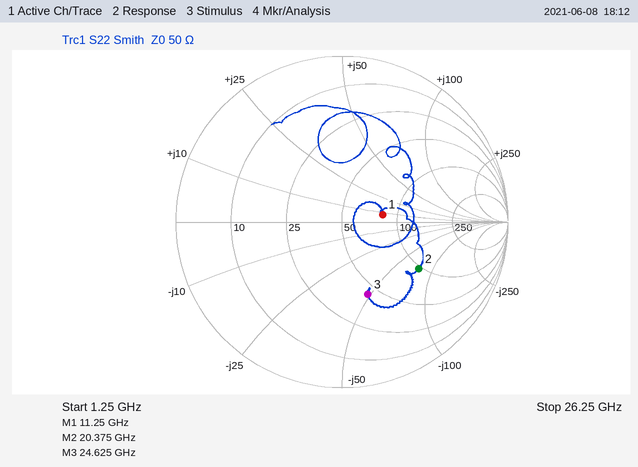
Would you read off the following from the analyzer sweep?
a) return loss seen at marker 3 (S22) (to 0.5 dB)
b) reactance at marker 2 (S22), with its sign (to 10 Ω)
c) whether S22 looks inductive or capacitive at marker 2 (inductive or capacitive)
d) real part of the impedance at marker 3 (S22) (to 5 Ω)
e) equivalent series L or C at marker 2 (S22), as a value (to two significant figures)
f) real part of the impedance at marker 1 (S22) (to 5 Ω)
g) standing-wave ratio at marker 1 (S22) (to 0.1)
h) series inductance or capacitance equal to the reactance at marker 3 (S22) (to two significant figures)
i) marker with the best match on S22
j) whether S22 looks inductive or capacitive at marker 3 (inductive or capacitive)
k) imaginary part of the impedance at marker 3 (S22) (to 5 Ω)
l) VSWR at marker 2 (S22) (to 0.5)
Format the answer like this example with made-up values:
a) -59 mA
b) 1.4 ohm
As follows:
a) 6.5 dB
b) -80 Ω
c) capacitive
d) 45 Ω
e) 100 fF
f) 80 Ω
g) 1.7
h) 130 fF
i) marker 1
j) capacitive
k) -50 Ω
l) 3.5
